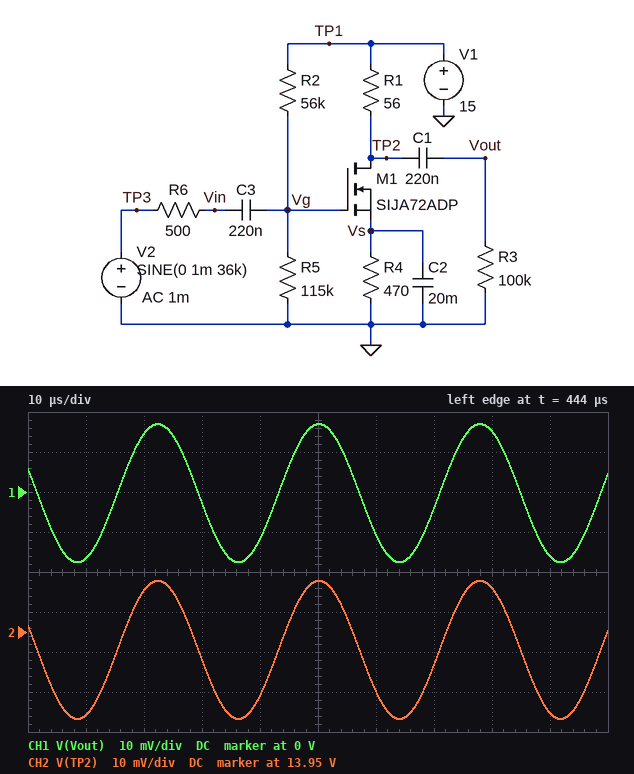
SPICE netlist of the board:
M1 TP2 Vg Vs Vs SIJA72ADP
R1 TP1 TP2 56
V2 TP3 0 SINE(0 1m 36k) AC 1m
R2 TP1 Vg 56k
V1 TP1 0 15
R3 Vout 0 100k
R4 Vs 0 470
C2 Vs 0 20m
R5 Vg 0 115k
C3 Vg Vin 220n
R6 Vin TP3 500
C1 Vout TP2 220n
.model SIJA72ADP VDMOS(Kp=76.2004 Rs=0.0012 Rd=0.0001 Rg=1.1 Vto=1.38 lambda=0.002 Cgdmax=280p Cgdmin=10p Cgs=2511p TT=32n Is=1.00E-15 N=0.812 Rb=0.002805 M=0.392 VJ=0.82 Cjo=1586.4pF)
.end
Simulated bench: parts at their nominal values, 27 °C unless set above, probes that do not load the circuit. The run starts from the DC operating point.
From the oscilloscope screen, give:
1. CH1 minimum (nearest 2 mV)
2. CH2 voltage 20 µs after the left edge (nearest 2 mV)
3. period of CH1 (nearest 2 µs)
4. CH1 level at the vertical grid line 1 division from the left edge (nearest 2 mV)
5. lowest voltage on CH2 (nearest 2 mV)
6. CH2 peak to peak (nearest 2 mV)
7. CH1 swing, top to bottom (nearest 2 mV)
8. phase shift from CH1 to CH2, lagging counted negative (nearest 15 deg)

-18 mV
13.960 V
28 µs
-16 mV
13.928 V
34 mV
34 mV
0 deg
